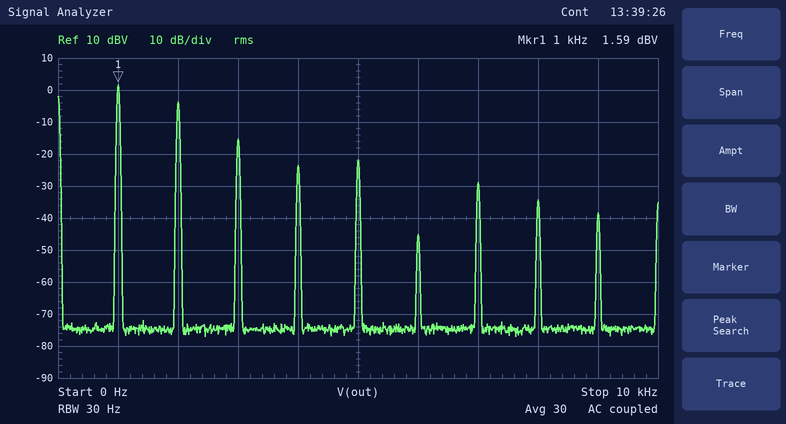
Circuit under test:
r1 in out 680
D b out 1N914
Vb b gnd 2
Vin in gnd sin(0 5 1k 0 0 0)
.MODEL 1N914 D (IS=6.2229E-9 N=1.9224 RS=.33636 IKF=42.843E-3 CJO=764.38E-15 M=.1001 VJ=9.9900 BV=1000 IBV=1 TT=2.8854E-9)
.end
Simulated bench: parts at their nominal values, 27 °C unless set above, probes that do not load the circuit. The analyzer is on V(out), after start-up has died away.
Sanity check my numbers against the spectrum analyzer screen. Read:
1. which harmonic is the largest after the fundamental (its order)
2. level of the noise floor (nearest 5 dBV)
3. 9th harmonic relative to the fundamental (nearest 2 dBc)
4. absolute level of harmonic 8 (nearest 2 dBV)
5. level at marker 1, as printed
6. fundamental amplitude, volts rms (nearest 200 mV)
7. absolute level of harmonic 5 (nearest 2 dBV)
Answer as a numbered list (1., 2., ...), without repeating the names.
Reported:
1. 2
2. -75 dBV
3. -40 dBc
4. -34 dBV
5. 1.59 dBV
6. 1.2 V
7. -22 dBV
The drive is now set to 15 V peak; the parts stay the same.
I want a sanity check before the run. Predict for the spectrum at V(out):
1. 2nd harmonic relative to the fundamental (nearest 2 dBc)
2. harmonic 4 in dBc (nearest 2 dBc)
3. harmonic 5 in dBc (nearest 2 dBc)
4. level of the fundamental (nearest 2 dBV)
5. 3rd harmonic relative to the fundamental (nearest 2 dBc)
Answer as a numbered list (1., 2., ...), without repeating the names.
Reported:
1. -6 dBc
2. -22 dBc
3. -32 dBc
4. 14 dBV
5. -28 dBc
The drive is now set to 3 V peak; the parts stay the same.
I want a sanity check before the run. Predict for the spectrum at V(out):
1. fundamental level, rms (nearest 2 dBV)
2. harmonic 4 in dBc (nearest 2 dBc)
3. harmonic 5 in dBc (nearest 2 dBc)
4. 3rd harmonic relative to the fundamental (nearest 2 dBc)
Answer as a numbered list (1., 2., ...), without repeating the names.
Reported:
1. -6 dBV
2. -28 dBc
3. -24 dBc
4. -12 dBc
